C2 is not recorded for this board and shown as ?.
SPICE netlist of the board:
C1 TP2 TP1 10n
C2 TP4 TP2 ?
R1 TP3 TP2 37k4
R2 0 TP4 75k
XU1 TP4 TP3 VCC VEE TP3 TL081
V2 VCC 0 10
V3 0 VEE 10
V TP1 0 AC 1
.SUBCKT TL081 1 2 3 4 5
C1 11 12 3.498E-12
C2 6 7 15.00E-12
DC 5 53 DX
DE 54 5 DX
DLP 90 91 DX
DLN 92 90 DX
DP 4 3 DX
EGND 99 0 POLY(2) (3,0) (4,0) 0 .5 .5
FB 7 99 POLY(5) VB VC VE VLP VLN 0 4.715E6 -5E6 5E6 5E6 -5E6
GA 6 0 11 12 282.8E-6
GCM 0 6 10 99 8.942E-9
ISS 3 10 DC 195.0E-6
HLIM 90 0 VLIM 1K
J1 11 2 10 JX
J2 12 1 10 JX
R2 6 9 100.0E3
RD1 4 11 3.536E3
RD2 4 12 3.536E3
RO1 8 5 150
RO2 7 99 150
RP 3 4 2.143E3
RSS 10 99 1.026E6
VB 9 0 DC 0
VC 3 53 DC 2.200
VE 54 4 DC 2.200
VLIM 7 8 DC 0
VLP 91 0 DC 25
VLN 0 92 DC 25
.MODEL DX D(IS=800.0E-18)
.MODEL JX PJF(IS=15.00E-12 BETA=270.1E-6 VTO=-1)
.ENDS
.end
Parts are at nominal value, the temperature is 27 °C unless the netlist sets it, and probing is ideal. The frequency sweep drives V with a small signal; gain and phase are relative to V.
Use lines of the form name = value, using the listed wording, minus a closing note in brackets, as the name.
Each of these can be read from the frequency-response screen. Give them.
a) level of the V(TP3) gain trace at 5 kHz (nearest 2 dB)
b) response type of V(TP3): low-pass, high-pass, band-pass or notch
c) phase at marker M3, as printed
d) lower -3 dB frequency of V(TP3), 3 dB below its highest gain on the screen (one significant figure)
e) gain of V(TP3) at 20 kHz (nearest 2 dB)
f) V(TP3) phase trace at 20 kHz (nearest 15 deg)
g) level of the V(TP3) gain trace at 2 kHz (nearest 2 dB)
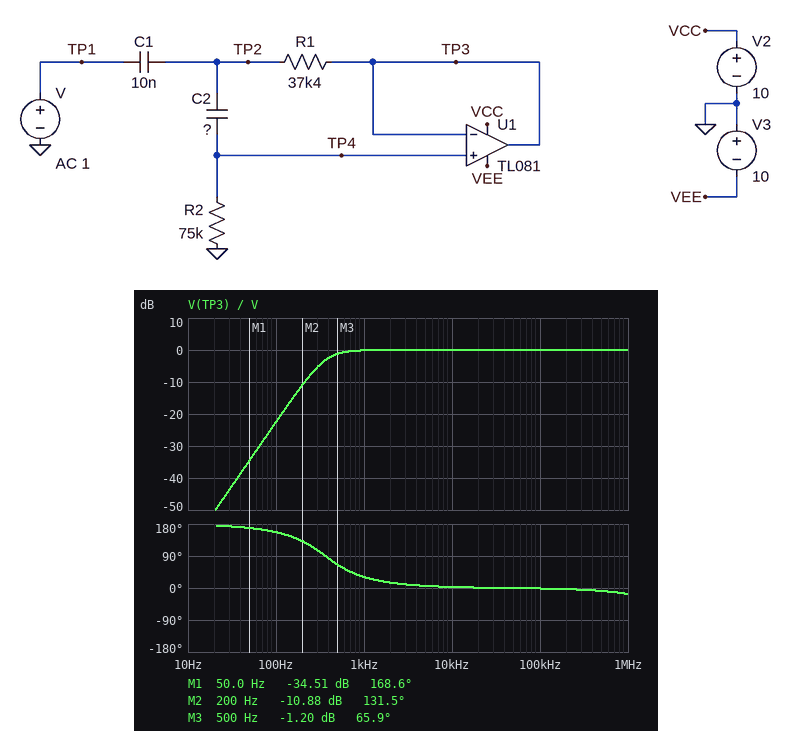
level of the V(TP3) gain trace at 5 kHz = 0 dB
response type of V(TP3): low-pass, high-pass, band-pass or notch = high-pass
phase at marker M3, as printed = 65.9 deg
lower -3 dB frequency of V(TP3), 3 dB below its highest gain on the screen = 400 Hz
gain of V(TP3) at 20 kHz = 0 dB
V(TP3) phase trace at 20 kHz = 0 deg
level of the V(TP3) gain trace at 2 kHz = 0 dB
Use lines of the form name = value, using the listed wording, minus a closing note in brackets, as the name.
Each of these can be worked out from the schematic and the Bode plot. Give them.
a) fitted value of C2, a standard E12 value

fitted value of C2, a standard E12 value = 6.8 nF
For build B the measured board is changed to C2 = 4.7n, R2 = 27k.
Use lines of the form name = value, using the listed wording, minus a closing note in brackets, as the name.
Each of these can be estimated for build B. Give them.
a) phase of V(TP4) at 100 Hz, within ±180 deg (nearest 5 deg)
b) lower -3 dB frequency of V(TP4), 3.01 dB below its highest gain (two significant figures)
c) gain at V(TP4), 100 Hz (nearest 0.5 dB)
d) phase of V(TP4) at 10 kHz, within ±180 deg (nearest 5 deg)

phase of V(TP4) at 100 Hz, within ±180 deg = 160 deg
lower -3 dB frequency of V(TP4), 3.01 dB below its highest gain = 1.6 kHz
gain at V(TP4), 100 Hz = -35.0 dB
phase of V(TP4) at 10 kHz, within ±180 deg = 10 deg
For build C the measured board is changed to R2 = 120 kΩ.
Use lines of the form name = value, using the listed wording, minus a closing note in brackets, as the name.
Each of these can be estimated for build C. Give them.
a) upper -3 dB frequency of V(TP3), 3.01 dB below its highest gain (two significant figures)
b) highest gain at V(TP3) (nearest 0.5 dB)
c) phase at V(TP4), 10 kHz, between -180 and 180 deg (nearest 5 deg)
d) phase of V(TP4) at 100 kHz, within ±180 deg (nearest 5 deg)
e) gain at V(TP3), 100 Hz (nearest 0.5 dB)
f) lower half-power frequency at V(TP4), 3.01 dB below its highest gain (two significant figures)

upper -3 dB frequency of V(TP3), 3.01 dB below its highest gain = 4.5 MHz
highest gain at V(TP3) = 0.5 dB
phase at V(TP4), 10 kHz, between -180 and 180 deg = 0 deg
phase of V(TP4) at 100 kHz, within ±180 deg = 0 deg
gain at V(TP3), 100 Hz = -18.0 dB
lower half-power frequency at V(TP4), 3.01 dB below its highest gain = 250 Hz
